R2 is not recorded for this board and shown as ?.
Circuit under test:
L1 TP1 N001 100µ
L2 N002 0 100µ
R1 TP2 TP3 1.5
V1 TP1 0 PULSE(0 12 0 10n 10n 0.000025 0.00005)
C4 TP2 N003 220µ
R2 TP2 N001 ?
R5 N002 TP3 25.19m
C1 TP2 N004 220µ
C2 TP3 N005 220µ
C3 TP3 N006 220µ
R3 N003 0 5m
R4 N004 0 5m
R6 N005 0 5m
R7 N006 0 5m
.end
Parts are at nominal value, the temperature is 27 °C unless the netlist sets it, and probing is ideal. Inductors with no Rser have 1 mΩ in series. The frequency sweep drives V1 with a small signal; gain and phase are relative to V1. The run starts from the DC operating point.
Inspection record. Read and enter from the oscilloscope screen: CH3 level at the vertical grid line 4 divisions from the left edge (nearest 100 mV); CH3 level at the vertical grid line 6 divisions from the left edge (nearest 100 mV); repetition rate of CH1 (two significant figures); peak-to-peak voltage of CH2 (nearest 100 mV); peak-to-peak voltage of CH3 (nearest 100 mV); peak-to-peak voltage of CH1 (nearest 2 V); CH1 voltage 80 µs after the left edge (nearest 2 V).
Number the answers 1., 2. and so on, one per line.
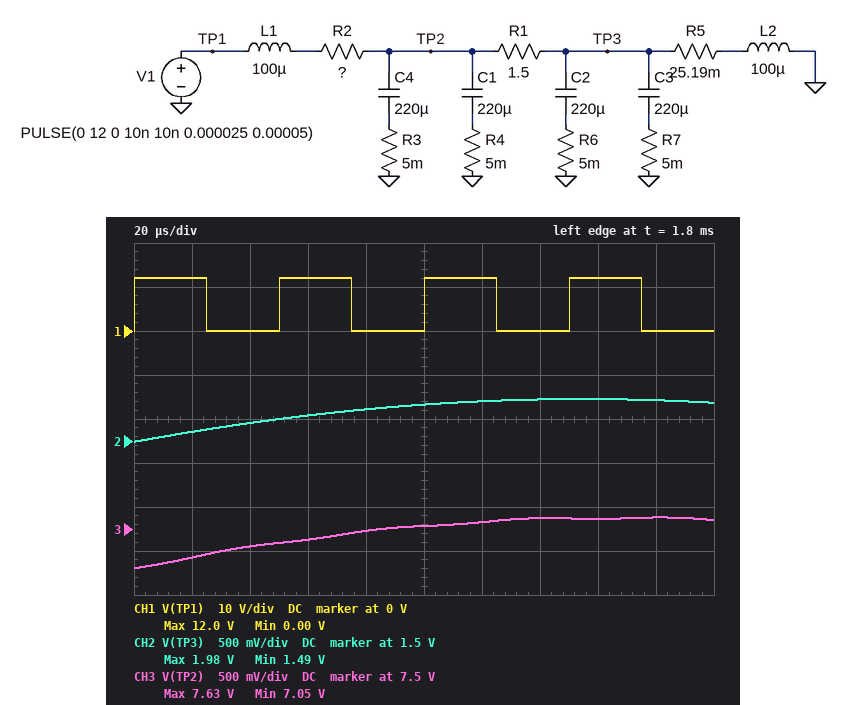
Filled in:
1. 7.5 V
2. 7.6 V
3. 20 kHz
4. 500 mV
5. 600 mV
6. 12 V
7. 0 V
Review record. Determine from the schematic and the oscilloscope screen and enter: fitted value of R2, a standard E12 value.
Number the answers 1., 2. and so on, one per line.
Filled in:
1. 0.056 Ω
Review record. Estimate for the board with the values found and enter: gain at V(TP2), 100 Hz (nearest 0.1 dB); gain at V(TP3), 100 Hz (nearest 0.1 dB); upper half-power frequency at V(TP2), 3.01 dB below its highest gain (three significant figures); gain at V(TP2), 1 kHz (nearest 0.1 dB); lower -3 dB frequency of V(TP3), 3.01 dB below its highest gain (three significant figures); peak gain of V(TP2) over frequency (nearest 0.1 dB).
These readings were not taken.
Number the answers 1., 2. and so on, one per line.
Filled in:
1. -0.2 dB
2. -27.1 dB
3. 792 Hz
4. -0.1 dB
5. 723 Hz
6. 15.1 dB
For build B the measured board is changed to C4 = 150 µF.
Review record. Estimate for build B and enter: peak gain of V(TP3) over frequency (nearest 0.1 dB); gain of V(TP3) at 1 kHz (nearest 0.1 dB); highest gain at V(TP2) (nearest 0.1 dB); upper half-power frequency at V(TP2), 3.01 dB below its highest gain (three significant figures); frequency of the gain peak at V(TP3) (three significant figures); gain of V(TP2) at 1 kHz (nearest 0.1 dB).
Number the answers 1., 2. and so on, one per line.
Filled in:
1. 13.2 dB
2. -4.0 dB
3. 14.8 dB
4. 829 Hz
5. 786 Hz
6. 2.4 dB
